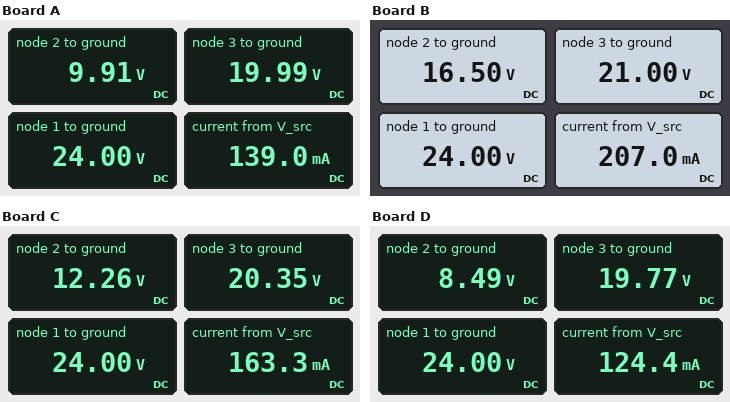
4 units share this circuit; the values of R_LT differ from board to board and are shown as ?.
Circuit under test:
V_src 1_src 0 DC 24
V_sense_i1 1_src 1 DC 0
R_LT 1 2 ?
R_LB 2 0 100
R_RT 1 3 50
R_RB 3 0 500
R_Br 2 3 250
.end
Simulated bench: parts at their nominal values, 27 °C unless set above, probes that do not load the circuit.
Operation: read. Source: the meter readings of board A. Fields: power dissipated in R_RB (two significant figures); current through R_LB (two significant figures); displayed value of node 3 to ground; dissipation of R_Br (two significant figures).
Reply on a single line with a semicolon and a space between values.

800 mW; 99 mA; 19.99 V; 410 mW
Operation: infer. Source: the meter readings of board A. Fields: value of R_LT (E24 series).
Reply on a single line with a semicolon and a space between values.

240 Ω
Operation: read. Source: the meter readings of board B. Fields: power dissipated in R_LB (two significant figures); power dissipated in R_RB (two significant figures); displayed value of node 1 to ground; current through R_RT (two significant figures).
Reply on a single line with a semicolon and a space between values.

2.7 W; 880 mW; 24.00 V; 60 mA
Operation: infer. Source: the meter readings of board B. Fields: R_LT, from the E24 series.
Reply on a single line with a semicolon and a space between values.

51 Ω
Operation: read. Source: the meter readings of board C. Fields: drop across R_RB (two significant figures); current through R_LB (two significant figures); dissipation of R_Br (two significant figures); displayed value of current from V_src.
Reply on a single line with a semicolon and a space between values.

20 V; 120 mA; 260 mW; 163.3 mA
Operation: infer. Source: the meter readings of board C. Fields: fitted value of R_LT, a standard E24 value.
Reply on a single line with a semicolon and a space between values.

130 Ω
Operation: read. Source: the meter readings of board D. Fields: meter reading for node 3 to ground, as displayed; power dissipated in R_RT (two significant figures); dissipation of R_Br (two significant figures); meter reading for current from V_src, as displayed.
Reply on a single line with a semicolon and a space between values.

19.77 V; 360 mW; 510 mW; 124.4 mA
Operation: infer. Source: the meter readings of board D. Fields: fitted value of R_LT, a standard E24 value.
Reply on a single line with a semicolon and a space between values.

390 Ω
